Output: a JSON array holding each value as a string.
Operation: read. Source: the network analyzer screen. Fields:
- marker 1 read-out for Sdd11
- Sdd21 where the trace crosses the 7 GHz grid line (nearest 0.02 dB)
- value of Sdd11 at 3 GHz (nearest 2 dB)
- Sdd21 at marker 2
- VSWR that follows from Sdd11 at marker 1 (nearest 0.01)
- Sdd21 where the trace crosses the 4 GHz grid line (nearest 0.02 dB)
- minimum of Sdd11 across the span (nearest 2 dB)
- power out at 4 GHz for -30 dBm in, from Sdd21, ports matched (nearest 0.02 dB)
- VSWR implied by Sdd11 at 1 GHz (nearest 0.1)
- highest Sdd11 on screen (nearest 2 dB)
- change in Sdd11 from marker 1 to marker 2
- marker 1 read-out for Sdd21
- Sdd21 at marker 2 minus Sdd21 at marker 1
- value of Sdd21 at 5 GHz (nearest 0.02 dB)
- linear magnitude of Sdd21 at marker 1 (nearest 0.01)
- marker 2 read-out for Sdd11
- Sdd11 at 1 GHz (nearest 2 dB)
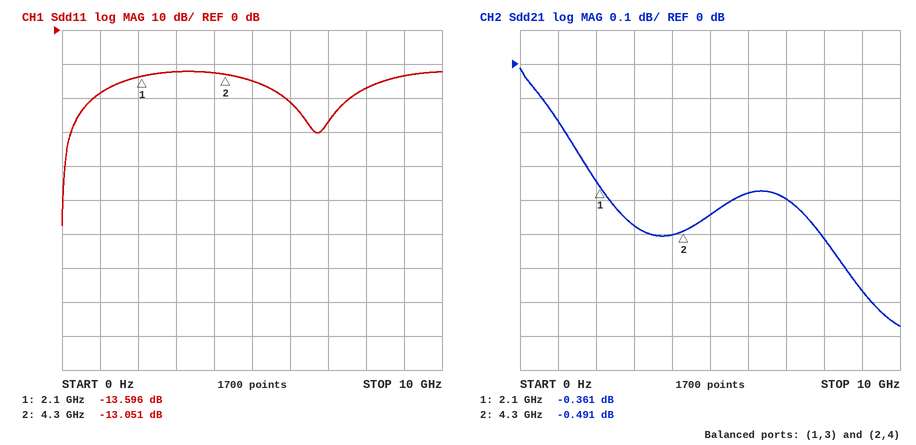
["-13.596 dB", "-0.40 dB", "-12 dB", "-0.491 dB", "1.53", "-0.50 dB", "-58 dB", "-30.50 dBm", "1.3", "-12 dB", "0.545 dB", "-0.361 dB", "-0.130 dB", "-0.44 dB", "0.96", "-13.051 dB", "-18 dB"]
